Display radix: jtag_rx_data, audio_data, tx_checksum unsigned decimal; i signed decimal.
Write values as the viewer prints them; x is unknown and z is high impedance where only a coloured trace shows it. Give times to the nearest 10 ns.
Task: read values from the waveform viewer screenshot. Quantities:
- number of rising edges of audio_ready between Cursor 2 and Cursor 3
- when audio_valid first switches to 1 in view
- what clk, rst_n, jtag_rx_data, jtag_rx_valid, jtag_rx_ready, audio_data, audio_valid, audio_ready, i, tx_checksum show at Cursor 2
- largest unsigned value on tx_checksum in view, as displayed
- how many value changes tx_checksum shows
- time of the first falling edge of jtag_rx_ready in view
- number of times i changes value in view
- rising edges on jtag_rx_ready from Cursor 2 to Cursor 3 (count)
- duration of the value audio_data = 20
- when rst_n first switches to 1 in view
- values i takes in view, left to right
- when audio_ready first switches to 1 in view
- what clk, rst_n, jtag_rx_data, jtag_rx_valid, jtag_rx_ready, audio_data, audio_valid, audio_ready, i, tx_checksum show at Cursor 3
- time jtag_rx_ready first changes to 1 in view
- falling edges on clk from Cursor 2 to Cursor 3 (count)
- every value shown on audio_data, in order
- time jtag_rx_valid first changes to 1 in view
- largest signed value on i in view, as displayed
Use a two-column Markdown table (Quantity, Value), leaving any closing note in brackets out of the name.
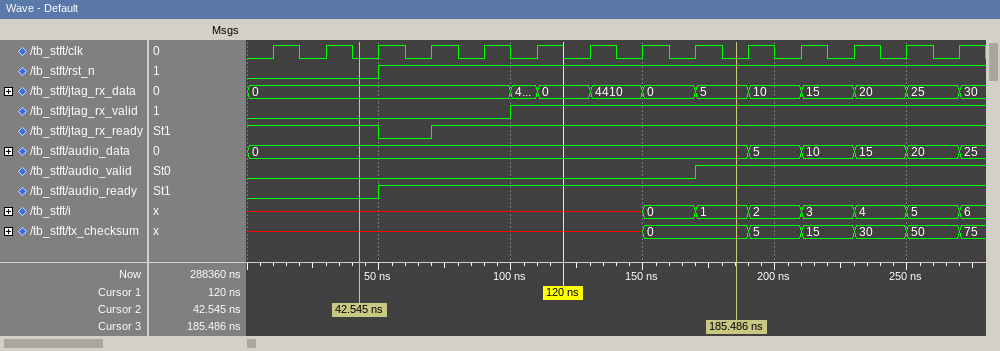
| Quantity | Value |
|---|---|
| number of rising edges of audio_ready between Cursor 2 and Cursor 3 | 1 |
| when audio_valid first switches to 1 in view | 170 ns |
| what clk, rst_n, jtag_rx_data, jtag_rx_valid, jtag_rx_ready, audio_data, audio_valid, audio_ready, i, tx_checksum show at Cursor 2 | clk=0, rst_n=0, jtag_rx_data=0, jtag_rx_valid=0, jtag_rx_ready=1, audio_data=0, audio_valid=0, audio_ready=0, i=x, tx_checksum=x |
| largest unsigned value on tx_checksum in view, as displayed | 75 |
| how many value changes tx_checksum shows | 6 |
| time of the first falling edge of jtag_rx_ready in view | 50 ns |
| number of times i changes value in view | 7 |
| rising edges on jtag_rx_ready from Cursor 2 to Cursor 3 | 1 |
| duration of the value audio_data = 20 | 20 ns |
| when rst_n first switches to 1 in view | 50 ns |
| values i takes in view, left to right | x, 0, 1, 2, 3, 4, 5, 6 |
| when audio_ready first switches to 1 in view | 50 ns |
| what clk, rst_n, jtag_rx_data, jtag_rx_valid, jtag_rx_ready, audio_data, audio_valid, audio_ready, i, tx_checksum show at Cursor 3 | clk=0, rst_n=1, jtag_rx_data=5, jtag_rx_valid=1, jtag_rx_ready=1, audio_data=0, audio_valid=1, audio_ready=1, i=1, tx_checksum=0 |
| time jtag_rx_ready first changes to 1 in view | 70 ns |
| falling edges on clk from Cursor 2 to Cursor 3 | 7 |
| every value shown on audio_data, in order | 0, 5, 10, 15, 20, 25 |
| time jtag_rx_valid first changes to 1 in view | 100 ns |
| largest signed value on i in view, as displayed | 6 |
